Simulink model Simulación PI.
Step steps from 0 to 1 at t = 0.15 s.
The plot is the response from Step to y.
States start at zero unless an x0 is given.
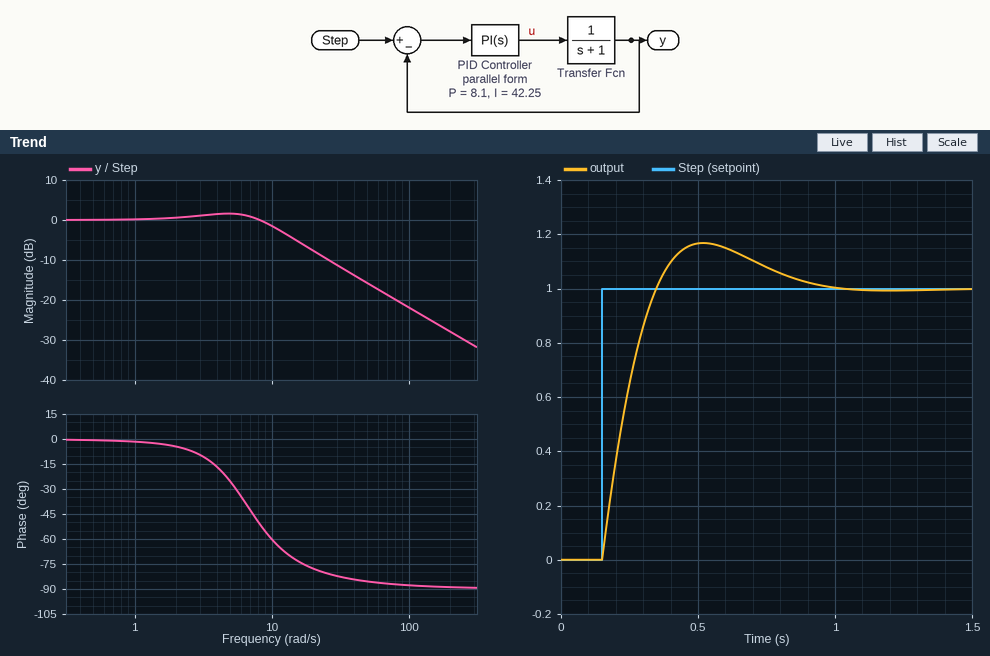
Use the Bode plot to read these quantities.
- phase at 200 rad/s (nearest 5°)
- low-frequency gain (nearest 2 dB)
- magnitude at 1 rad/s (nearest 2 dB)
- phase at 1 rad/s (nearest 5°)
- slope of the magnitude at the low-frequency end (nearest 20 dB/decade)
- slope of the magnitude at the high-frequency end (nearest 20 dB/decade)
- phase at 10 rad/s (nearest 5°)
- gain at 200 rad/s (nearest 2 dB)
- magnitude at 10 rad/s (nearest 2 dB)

-90°
0 dB
0 dB
0°
0 dB/decade
-20 dB/decade
-60°
-28 dB
-2 dB
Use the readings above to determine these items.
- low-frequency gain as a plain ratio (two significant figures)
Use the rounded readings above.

1.0
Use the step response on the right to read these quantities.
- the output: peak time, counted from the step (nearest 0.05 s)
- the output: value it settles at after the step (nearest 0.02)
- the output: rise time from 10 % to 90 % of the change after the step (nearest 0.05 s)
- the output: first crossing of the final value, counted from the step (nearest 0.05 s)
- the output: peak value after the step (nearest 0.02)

0.35 s
1.00
0.15 s
0.20 s
1.16
